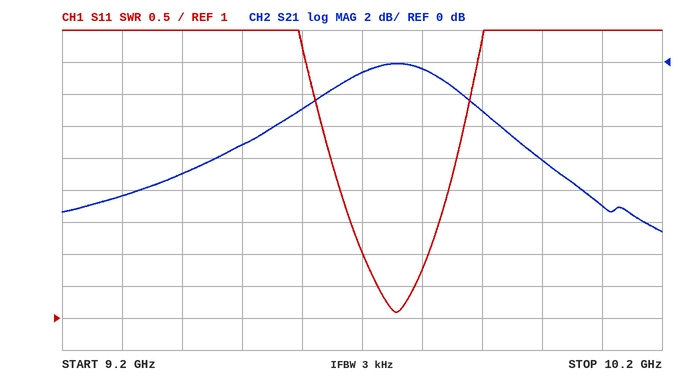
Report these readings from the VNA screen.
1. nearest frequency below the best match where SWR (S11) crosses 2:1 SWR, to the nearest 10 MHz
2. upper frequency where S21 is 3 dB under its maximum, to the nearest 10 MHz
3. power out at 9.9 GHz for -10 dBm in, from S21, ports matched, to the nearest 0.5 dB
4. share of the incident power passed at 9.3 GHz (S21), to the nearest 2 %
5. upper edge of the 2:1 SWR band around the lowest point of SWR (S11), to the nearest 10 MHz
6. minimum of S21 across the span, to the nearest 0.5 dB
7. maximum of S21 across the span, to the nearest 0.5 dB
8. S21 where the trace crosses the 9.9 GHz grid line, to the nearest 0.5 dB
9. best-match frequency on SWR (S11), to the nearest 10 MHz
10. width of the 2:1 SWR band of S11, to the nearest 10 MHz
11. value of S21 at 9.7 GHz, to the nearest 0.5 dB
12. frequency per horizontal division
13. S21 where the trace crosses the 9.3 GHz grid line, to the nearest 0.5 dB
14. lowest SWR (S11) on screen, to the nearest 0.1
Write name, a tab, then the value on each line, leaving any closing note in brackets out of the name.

nearest frequency below the best match where SWR (S11) crosses 2:1 SWR, to the nearest 10 MHz	9.70 GHz
upper frequency where S21 is 3 dB under its maximum, to the nearest 10 MHz	9.90 GHz
power out at 9.9 GHz for -10 dBm in, from S21, ports matched, to the nearest 0.5 dB	-13.0 dBm
share of the incident power passed at 9.3 GHz (S21), to the nearest 2 %	14 %
upper edge of the 2:1 SWR band around the lowest point of SWR (S11), to the nearest 10 MHz	9.81 GHz
minimum of S21 across the span, to the nearest 0.5 dB	-10.5 dB
maximum of S21 across the span, to the nearest 0.5 dB	0.0 dB
S21 where the trace crosses the 9.9 GHz grid line, to the nearest 0.5 dB	-3.0 dB
best-match frequency on SWR (S11), to the nearest 10 MHz	9.76 GHz
width of the 2:1 SWR band of S11, to the nearest 10 MHz	110 MHz
value of S21 at 9.7 GHz, to the nearest 0.5 dB	-0.5 dB
frequency per horizontal division	100 MHz
S21 where the trace crosses the 9.3 GHz grid line, to the nearest 0.5 dB	-8.5 dB
lowest SWR (S11) on screen, to the nearest 0.1	1.1
